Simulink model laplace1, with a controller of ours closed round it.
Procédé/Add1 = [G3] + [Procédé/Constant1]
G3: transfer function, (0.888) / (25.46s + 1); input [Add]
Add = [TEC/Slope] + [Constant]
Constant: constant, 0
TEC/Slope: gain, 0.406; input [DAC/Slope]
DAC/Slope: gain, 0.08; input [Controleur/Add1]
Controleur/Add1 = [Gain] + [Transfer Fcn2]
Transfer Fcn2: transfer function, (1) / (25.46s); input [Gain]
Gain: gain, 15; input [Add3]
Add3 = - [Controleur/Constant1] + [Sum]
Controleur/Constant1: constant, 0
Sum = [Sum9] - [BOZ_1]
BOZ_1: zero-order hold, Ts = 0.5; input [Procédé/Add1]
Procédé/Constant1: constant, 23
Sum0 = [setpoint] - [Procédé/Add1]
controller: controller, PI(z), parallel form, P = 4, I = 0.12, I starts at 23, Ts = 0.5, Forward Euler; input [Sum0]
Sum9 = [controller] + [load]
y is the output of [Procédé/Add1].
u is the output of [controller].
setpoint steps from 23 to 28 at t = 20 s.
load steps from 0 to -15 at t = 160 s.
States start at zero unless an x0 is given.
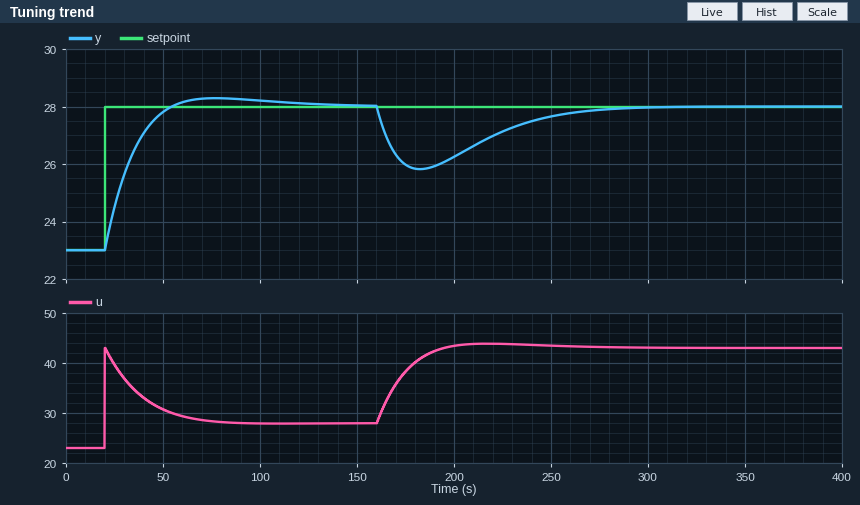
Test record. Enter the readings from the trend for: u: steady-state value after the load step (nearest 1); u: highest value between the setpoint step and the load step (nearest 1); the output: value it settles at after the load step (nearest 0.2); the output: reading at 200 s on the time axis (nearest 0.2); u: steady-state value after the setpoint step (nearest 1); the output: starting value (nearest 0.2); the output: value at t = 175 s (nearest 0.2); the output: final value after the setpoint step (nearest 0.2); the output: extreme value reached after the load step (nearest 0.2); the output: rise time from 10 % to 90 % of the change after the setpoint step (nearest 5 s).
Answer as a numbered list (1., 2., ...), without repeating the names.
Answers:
1. 43
2. 43
3. 28.0
4. 26.2
5. 28
6. 23.0
7. 26.0
8. 28.0
9. 25.8
10. 25 s
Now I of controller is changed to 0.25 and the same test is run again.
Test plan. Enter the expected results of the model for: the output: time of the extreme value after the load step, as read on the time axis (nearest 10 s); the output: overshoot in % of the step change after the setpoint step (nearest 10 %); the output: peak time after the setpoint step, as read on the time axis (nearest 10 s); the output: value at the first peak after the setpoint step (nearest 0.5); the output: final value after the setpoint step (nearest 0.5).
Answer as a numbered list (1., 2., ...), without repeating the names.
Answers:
1. 180 s
2. 20 %
3. 60 s
4. 29.0
5. 28.0
